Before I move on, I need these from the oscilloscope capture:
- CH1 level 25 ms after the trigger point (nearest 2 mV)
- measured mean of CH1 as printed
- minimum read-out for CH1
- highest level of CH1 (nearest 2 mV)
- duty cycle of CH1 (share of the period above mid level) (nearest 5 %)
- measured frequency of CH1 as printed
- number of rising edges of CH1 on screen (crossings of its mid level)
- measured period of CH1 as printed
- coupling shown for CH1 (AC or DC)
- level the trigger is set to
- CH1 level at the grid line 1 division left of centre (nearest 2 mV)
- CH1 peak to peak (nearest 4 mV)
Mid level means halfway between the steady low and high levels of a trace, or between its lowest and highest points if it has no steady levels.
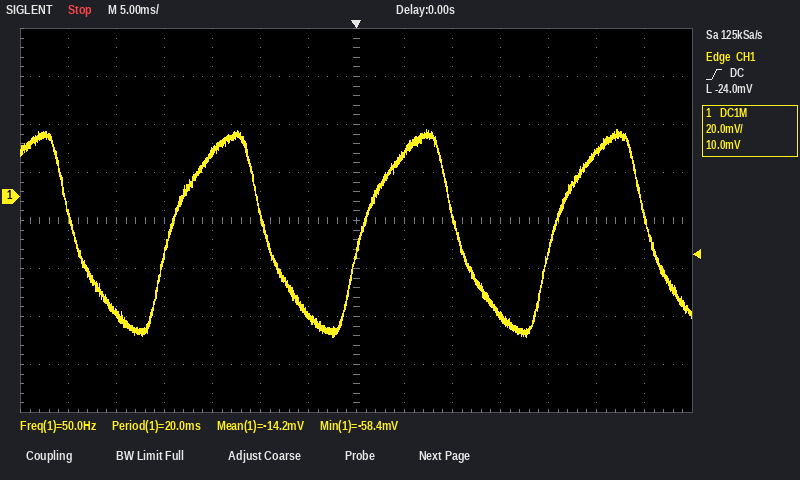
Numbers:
18 mV
-14.2 mV
-58.4 mV
28 mV
50 %
50.0 Hz
3
20.0 ms
DC
-24.0 mV
-50 mV
88 mV
